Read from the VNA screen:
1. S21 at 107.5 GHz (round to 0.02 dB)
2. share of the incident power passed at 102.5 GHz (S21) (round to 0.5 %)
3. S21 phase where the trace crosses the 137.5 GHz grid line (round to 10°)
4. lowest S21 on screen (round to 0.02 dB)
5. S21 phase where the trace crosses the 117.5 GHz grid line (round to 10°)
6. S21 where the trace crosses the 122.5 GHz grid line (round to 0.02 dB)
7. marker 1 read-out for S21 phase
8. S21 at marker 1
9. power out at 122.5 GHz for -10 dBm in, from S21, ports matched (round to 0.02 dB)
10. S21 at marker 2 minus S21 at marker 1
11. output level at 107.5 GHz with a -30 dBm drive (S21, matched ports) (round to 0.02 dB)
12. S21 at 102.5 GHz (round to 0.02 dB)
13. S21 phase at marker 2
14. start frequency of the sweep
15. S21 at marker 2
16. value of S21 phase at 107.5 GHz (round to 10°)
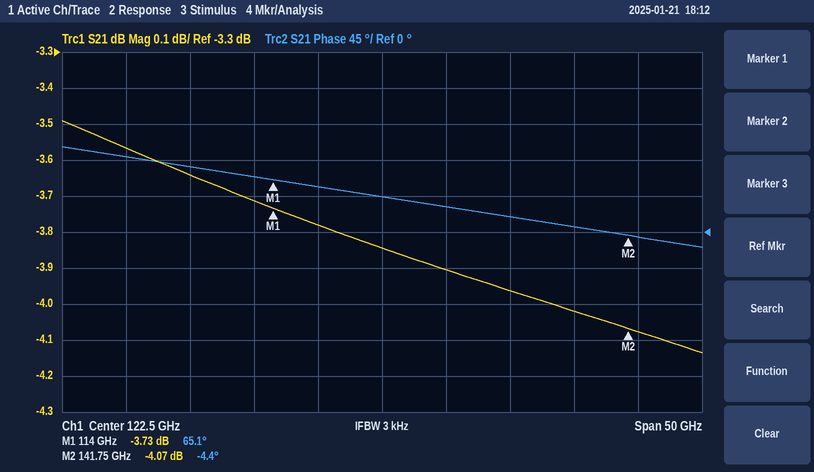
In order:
-3.64 dB
44.0 %
10°
-4.14 dB
60°
-3.84 dB
65.1°
-3.73 dB
-13.84 dBm
-0.34 dB
-33.64 dBm
-3.56 dB
-4.4°
97.5 GHz
-4.07 dB
80°
